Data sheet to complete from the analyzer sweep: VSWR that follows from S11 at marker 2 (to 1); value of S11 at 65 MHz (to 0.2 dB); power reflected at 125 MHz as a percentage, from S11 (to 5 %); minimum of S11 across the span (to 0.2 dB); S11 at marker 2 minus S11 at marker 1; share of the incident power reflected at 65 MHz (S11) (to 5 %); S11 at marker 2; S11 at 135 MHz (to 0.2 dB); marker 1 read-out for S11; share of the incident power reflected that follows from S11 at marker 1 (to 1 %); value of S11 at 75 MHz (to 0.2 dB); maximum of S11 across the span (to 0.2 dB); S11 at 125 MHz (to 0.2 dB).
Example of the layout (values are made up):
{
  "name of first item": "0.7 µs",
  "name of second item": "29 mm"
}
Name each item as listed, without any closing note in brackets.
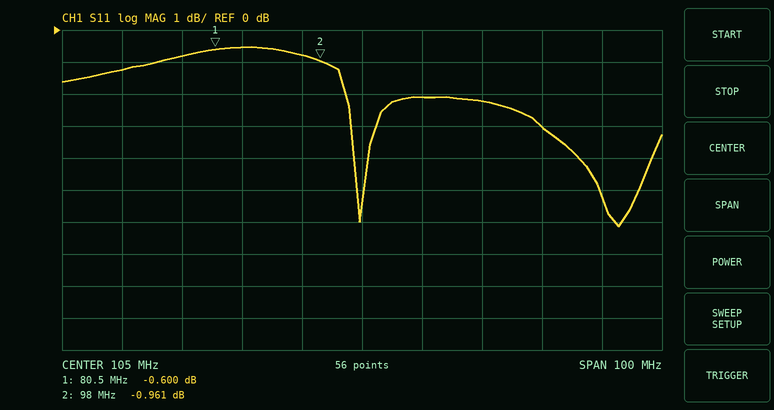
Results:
{
  "VSWR that follows from S11 at marker 2": "18",
  "value of S11 at 65 MHz": "-1.2 dB",
  "power reflected at 125 MHz as a percentage, from S11": "60 %",
  "minimum of S11 across the span": "-6.2 dB",
  "S11 at marker 2 minus S11 at marker 1": "-0.361 dB",
  "share of the incident power reflected at 65 MHz (S11)": "75 %",
  "S11 at marker 2": "-0.961 dB",
  "S11 at 135 MHz": "-3.0 dB",
  "marker 1 read-out for S11": "-0.600 dB",
  "share of the incident power reflected that follows from S11 at marker 1": "87 %",
  "value of S11 at 75 MHz": "-0.8 dB",
  "maximum of S11 across the span": "-0.6 dB",
  "S11 at 125 MHz": "-2.2 dB"
}
